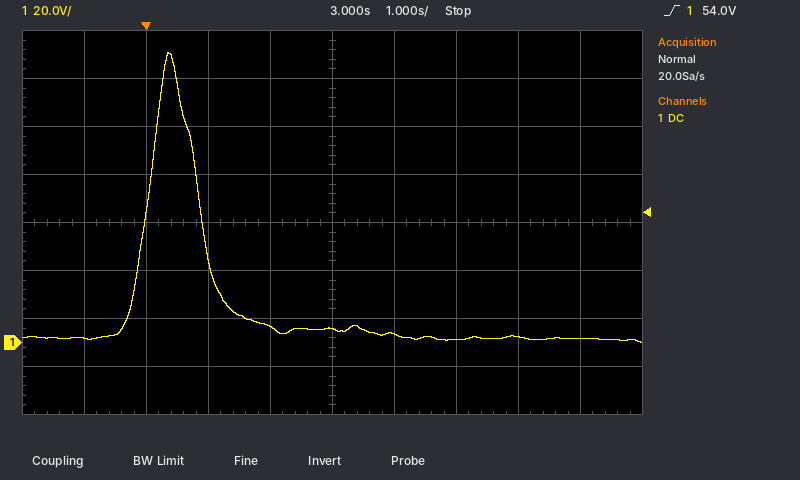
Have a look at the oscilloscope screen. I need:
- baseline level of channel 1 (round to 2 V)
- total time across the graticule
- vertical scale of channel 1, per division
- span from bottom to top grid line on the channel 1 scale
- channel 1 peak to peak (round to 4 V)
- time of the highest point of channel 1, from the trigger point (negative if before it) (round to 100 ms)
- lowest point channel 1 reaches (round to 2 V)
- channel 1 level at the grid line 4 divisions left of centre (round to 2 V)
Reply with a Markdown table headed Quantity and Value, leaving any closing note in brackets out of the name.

| Quantity | Value |
|---|---|
| baseline level of channel 1 | 2 V |
| total time across the graticule | 10 s |
| vertical scale of channel 1, per division | 20 V |
| span from bottom to top grid line on the channel 1 scale | 160 V |
| channel 1 peak to peak | 120 V |
| time of the highest point of channel 1, from the trigger point (negative if before it) | +400 ms |
| lowest point channel 1 reaches | 0 V |
| channel 1 level at the grid line 4 divisions left of centre | 2 V |
